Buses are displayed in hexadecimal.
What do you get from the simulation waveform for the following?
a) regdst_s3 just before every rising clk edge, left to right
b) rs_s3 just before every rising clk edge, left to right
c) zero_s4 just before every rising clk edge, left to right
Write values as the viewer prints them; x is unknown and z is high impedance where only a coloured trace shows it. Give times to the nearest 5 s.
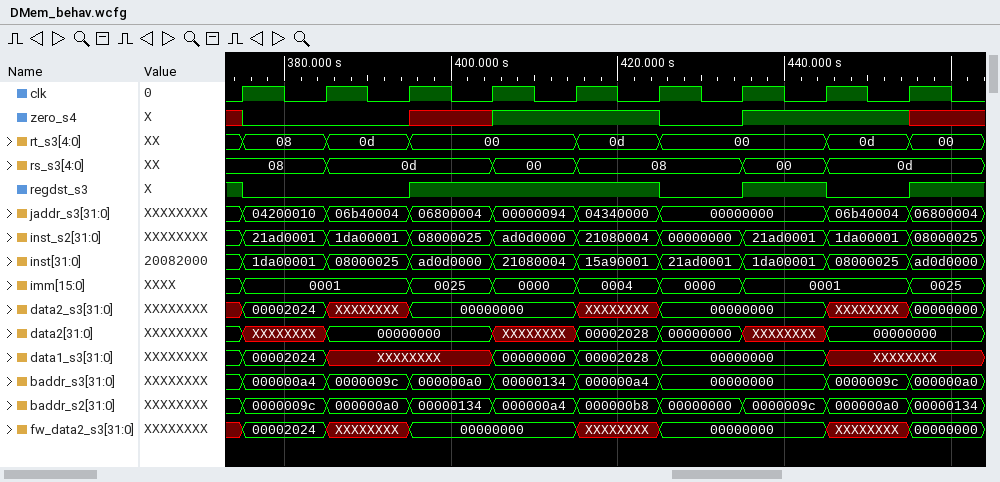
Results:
1 0 0 1 1 1 0 1 0
08, 08, 0d, 0d, 00, 08, 08, 00, 0d
x 0 0 x 1 1 0 1 1
